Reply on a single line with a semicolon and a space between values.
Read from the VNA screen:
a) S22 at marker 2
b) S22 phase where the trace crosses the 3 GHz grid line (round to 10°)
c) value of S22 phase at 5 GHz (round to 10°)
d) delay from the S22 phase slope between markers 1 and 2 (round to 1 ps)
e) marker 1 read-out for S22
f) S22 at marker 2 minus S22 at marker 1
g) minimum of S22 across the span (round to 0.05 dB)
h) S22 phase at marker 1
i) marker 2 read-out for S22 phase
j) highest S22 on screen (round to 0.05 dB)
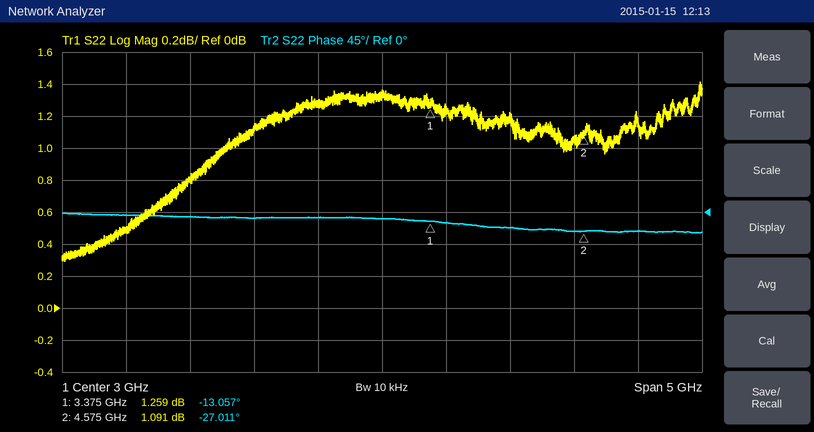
1.091 dB; -10°; -30°; 32 ps; 1.259 dB; -0.168 dB; 0.30 dB; -13.057°; -27.011°; 1.40 dB
